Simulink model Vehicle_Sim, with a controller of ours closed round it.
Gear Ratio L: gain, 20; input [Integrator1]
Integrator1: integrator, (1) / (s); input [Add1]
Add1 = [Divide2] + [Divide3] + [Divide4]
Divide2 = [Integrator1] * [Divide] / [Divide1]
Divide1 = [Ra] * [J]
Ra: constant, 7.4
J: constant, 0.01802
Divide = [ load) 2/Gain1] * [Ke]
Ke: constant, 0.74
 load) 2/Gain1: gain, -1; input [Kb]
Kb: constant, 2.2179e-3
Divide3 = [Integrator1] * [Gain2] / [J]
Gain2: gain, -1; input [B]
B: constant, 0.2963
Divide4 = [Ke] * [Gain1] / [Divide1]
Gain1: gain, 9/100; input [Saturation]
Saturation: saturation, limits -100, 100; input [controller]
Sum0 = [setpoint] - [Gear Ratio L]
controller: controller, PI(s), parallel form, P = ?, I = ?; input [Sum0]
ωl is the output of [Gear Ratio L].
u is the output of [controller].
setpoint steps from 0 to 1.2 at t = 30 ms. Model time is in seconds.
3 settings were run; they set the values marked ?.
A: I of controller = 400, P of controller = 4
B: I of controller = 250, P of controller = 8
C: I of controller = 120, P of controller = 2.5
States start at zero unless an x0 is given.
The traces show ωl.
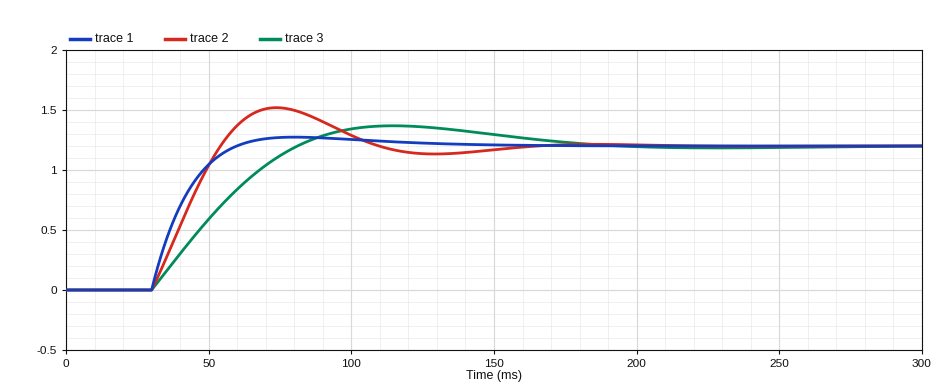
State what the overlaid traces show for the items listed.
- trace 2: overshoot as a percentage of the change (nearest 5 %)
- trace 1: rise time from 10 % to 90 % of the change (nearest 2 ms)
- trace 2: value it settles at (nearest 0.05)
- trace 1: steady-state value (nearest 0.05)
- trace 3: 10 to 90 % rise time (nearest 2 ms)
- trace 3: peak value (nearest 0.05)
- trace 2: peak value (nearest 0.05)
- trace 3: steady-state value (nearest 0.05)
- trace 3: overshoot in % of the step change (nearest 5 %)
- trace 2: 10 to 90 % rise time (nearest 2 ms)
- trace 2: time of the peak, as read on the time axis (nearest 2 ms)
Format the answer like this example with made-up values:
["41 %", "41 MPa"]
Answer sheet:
["25 %", "20 ms", "1.20", "1.20", "38 ms", "1.35", "1.50", "1.20", "15 %", "18 ms", "74 ms"]
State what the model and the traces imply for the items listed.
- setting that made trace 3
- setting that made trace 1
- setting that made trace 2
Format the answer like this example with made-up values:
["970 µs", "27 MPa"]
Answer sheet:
["C", "B", "A"]
